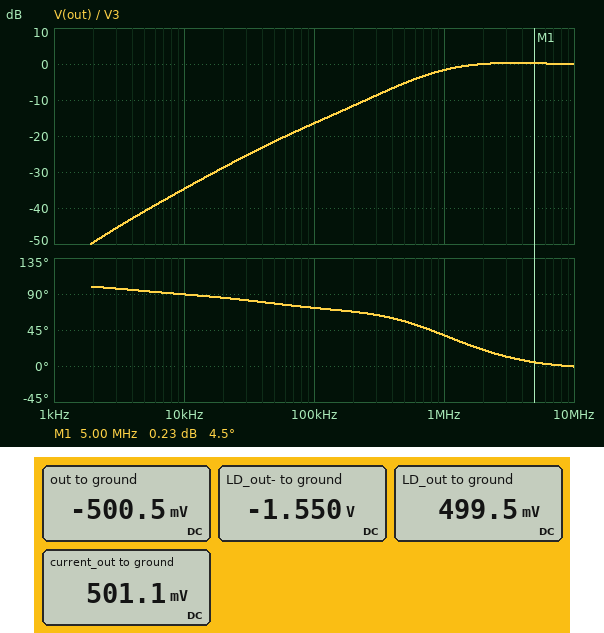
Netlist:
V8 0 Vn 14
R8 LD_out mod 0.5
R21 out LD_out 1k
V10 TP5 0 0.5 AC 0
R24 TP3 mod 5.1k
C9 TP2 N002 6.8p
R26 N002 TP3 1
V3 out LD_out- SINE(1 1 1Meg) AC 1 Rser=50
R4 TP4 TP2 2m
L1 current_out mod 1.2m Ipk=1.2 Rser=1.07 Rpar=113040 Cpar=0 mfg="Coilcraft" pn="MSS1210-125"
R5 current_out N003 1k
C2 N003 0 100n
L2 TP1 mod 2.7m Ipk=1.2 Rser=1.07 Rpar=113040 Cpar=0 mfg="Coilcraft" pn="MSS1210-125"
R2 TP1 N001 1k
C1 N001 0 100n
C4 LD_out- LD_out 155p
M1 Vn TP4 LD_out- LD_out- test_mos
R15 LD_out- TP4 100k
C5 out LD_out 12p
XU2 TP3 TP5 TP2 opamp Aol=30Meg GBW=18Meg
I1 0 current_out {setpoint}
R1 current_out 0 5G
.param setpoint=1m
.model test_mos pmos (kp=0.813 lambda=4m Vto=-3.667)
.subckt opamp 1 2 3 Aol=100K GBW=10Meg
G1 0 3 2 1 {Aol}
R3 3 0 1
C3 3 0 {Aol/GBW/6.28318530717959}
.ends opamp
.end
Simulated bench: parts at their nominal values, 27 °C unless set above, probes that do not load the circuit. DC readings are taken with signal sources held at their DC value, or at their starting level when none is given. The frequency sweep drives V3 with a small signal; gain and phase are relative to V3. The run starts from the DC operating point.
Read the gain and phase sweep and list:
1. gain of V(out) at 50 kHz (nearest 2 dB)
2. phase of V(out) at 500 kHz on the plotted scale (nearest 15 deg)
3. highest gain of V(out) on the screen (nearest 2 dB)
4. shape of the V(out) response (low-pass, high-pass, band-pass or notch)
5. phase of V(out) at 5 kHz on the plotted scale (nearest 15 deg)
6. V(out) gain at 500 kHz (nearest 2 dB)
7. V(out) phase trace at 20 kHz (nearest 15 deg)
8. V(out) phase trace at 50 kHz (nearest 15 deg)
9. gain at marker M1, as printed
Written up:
-22 dB
60 deg
0 dB
high-pass
90 deg
-6 dB
90 deg
75 deg
0.23 dB
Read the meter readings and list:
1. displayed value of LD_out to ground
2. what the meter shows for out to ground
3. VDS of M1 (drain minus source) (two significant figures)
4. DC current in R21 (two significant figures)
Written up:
499.5 mV
-500.5 mV
-12 V
1.0 mA
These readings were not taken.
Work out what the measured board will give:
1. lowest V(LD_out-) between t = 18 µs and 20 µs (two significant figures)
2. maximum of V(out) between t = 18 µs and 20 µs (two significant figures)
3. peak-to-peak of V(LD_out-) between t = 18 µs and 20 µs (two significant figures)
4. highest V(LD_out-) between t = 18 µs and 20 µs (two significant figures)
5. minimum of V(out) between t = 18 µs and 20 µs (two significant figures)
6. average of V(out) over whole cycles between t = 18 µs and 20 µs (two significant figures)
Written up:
-2.2 V
320 mV
1.3 V
-920 mV
-1.3 V
-500 mV
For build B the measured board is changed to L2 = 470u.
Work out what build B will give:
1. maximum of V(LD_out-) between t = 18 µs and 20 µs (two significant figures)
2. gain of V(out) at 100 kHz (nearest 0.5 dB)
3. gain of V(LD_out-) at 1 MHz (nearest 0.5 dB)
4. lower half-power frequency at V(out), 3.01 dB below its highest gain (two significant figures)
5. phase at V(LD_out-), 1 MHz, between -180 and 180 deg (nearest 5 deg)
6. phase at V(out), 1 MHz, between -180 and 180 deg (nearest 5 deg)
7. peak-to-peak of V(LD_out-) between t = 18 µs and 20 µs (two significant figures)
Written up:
-940 mV
-15.5 dB
-4.5 dB
820 kHz
125 deg
35 deg
1.2 V
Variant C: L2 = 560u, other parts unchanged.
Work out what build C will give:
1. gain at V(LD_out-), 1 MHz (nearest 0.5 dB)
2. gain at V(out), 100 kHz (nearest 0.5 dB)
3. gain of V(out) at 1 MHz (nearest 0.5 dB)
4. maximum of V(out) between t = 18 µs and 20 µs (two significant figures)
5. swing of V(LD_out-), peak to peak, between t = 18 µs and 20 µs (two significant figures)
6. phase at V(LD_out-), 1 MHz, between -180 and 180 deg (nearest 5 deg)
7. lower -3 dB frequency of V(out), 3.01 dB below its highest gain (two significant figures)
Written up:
-4.5 dB
-15.5 dB
-2.0 dB
310 mV
1.2 V
125 deg
820 kHz
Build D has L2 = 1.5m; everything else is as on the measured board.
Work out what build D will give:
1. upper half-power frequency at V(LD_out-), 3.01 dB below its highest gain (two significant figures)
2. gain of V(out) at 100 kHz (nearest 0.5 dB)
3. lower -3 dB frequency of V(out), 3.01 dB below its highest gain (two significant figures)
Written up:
780 kHz
-16.0 dB
800 kHz
